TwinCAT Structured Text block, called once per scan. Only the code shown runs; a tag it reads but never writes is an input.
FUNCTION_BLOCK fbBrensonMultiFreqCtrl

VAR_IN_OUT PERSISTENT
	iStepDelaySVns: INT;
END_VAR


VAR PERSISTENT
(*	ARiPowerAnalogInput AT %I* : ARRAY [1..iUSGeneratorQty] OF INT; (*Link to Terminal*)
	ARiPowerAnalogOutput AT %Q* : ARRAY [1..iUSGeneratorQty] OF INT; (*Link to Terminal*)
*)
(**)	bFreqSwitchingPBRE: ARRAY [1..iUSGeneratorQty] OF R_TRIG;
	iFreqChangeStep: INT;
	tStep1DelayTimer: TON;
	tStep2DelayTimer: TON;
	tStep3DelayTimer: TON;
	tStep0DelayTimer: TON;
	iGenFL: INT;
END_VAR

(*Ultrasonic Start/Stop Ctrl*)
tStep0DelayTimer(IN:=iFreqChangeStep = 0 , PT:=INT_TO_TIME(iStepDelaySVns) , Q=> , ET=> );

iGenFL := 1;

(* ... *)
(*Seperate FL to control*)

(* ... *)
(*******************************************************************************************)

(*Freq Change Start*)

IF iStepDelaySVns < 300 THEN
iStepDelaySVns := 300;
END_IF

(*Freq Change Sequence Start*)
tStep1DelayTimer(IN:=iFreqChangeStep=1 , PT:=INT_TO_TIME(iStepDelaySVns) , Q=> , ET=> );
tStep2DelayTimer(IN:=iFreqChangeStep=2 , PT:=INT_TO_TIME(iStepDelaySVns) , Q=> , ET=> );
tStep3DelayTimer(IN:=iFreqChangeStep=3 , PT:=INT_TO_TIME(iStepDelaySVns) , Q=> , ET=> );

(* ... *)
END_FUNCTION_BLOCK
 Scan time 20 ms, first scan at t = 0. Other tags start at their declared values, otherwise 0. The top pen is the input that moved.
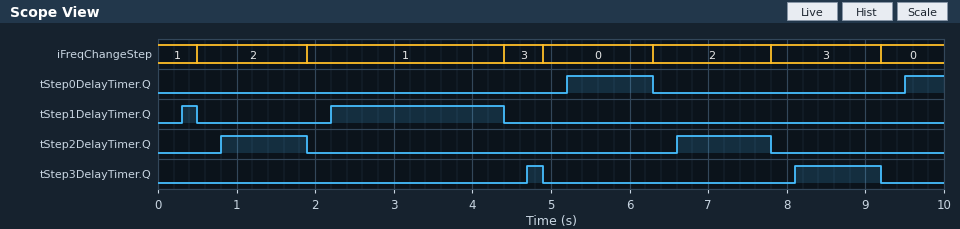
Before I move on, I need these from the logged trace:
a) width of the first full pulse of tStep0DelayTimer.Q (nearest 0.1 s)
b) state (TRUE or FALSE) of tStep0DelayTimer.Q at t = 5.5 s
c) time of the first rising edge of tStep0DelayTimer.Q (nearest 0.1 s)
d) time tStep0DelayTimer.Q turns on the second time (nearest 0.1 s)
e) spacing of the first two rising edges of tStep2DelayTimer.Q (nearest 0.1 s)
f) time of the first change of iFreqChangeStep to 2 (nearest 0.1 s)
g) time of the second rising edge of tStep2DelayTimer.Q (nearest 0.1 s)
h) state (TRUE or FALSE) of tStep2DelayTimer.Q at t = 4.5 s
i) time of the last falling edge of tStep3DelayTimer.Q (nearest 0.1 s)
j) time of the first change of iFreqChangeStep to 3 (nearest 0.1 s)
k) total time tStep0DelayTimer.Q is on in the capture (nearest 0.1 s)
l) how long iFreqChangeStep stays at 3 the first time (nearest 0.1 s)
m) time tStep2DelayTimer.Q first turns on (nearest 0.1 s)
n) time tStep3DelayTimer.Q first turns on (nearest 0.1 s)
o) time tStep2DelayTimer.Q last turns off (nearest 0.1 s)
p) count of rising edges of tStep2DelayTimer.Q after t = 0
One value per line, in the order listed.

1.1 s
TRUE
5.2 s
9.5 s
5.8 s
0.5 s
6.6 s
FALSE
9.2 s
4.4 s
1.6 s
0.5 s
0.8 s
4.7 s
7.8 s
2
